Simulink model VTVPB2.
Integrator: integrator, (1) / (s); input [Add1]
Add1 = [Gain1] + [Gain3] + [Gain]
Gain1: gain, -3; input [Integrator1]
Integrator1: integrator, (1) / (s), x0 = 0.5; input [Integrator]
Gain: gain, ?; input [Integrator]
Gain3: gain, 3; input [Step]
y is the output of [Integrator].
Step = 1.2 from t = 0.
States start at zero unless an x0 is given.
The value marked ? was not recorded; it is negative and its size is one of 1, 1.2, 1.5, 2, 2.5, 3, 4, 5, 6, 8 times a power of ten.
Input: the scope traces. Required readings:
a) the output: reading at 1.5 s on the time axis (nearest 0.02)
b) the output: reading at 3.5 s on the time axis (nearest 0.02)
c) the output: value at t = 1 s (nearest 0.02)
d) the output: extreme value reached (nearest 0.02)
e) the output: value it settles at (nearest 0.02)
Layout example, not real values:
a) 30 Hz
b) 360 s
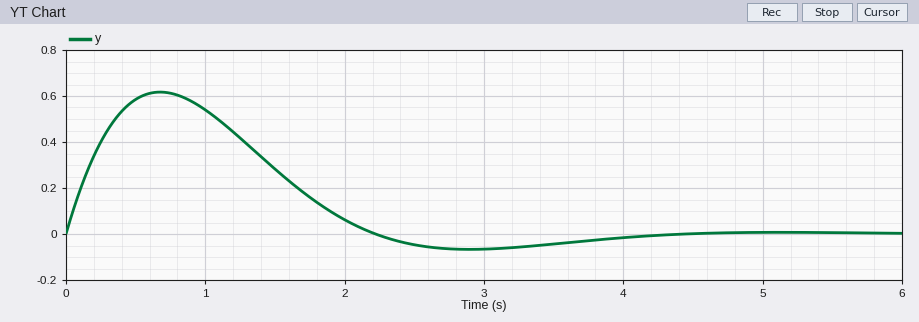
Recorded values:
a) 0.28
b) -0.04
c) 0.54
d) 0.62
e) 0.00
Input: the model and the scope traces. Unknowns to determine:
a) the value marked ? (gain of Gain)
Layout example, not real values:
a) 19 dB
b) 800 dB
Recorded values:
a) -2
